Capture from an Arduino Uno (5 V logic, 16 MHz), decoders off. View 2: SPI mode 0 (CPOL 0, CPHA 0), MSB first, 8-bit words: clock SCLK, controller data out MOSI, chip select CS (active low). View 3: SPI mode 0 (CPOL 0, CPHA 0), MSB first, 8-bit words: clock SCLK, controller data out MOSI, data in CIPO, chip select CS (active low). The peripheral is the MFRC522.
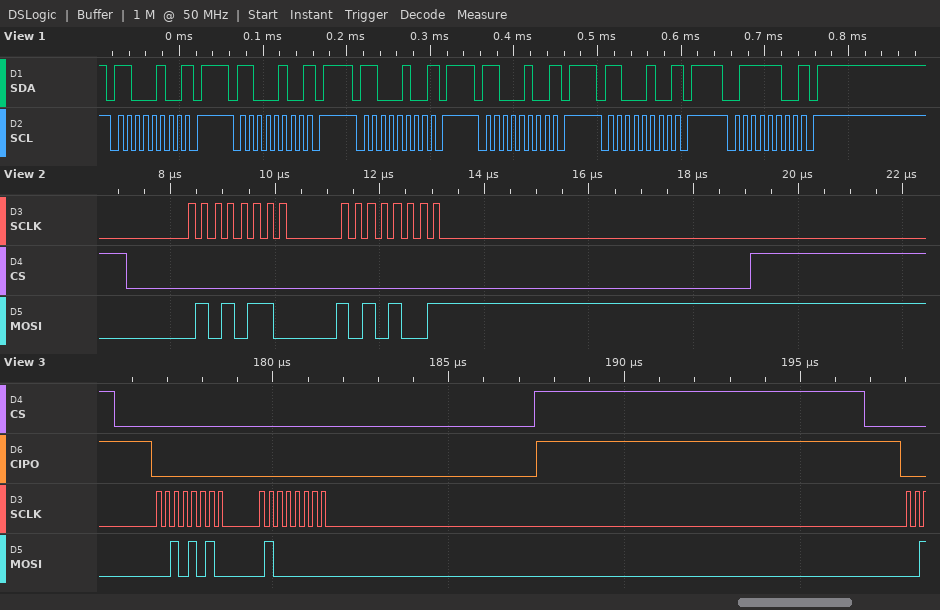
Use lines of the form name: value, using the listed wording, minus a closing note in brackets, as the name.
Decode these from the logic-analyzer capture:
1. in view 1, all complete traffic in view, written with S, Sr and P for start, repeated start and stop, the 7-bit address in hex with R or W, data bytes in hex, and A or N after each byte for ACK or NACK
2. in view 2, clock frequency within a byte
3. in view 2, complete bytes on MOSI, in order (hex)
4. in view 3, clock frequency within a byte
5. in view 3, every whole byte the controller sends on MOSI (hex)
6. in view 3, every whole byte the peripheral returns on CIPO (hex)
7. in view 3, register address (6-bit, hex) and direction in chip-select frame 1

in view 1, all complete traffic in view, written with S, Sr and P for start, repeated start and stop, the 7-bit address in hex with R or W, data bytes in hex, and A or N after each byte for ACK or NACK: S 62W N P S 62W N P S 62W N P S 62W N P S 62W N P S 3EW N P
in view 2, clock frequency within a byte: 4 MHz
in view 2, complete bytes on MOSI, in order: 56 A9
in view 3, clock frequency within a byte: 4 MHz
in view 3, every whole byte the controller sends on MOSI: 2A 40
in view 3, every whole byte the peripheral returns on CIPO: 00 00
in view 3, register address (6-bit, hex) and direction in chip-select frame 1: 0x15 write
